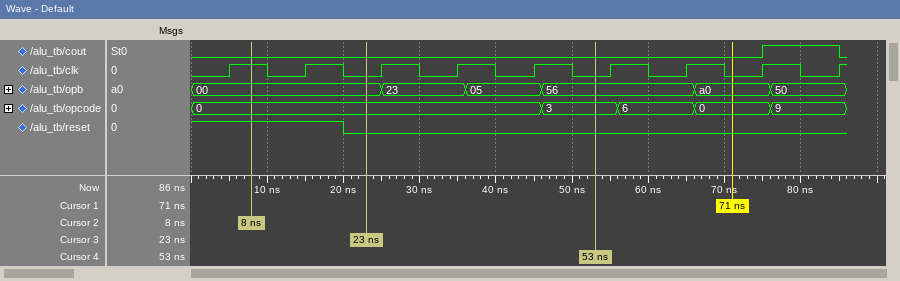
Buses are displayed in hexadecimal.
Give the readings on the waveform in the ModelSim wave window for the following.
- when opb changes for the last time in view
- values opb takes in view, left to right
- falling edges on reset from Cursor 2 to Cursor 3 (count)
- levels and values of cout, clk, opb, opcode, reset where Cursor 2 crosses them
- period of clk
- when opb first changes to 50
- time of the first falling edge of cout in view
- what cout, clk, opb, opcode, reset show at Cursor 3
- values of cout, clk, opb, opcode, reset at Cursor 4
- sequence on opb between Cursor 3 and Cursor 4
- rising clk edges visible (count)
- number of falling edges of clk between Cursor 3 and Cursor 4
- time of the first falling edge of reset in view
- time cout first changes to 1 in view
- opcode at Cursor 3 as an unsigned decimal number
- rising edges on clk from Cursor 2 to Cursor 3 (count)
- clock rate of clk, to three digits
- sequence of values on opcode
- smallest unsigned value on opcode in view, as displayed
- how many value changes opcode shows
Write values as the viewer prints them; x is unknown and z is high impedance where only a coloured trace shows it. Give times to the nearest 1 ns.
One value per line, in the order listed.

76 ns
00, 23, 05, 56, a0, 50
1
cout=0, clk=1, opb=00, opcode=0, reset=1
10 ns
76 ns
85 ns
cout=0, clk=0, opb=00, opcode=0, reset=0
cout=0, clk=0, opb=56, opcode=3, reset=0
00, 23, 05, 56
9
3
20 ns
75 ns
0
1
100 MHz
0, 3, 6, 0, 9
0
4
